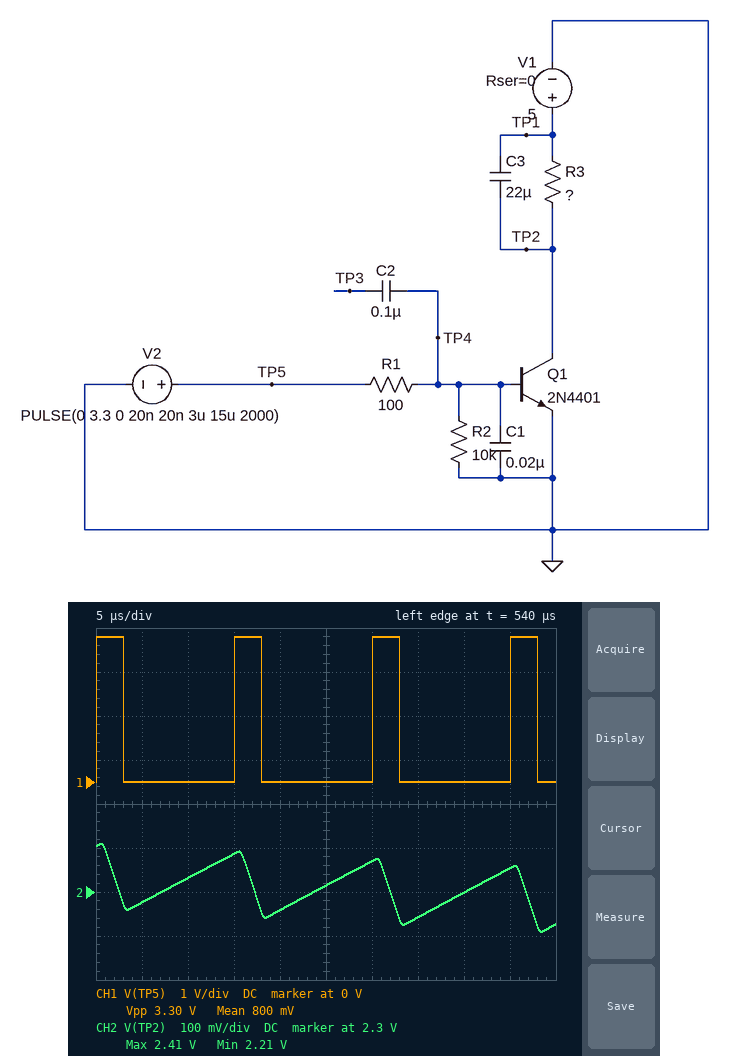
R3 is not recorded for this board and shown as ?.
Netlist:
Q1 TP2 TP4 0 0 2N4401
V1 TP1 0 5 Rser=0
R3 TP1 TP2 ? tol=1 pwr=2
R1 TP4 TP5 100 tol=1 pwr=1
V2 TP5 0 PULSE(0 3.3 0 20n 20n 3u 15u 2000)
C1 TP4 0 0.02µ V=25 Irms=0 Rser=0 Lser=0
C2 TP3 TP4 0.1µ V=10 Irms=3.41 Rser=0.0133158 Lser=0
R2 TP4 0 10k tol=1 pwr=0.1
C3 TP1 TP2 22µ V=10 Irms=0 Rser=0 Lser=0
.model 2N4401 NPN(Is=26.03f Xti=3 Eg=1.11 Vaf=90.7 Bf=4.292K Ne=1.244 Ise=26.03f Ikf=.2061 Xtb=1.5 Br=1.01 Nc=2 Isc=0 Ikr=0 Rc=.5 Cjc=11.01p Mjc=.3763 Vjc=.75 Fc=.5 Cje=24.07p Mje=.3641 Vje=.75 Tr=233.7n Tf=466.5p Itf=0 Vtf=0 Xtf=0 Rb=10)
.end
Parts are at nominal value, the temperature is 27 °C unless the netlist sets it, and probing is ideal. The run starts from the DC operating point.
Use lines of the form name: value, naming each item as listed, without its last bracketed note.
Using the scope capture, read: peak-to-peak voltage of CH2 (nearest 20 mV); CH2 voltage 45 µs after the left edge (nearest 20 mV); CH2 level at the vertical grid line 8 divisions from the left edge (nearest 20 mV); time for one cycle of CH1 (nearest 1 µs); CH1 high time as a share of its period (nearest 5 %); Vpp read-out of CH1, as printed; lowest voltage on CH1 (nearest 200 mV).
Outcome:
peak-to-peak voltage of CH2: 200 mV
CH2 voltage 45 µs after the left edge: 2.36 V
CH2 level at the vertical grid line 8 divisions from the left edge: 2.30 V
time for one cycle of CH1: 15 µs
CH1 high time as a share of its period: 20 %
Vpp read-out of CH1, as printed: 3.30 V
lowest voltage on CH1: 0 V
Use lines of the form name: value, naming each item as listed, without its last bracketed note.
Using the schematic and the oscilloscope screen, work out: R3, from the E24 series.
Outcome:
R3, from the E24 series: 11 Ω
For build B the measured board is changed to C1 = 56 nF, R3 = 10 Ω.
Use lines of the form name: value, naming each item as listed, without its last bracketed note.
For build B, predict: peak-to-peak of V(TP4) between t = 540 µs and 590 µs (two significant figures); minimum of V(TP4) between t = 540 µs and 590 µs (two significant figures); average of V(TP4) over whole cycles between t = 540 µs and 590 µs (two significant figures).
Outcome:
peak-to-peak of V(TP4) between t = 540 µs and 590 µs: 970 mV
minimum of V(TP4) between t = 540 µs and 590 µs: 110 mV
average of V(TP4) over whole cycles between t = 540 µs and 590 µs: 460 mV
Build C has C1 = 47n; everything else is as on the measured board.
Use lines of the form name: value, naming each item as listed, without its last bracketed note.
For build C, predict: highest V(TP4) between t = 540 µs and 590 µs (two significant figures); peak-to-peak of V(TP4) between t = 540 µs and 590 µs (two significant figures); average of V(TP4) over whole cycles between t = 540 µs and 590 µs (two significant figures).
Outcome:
highest V(TP4) between t = 540 µs and 590 µs: 1.1 V
peak-to-peak of V(TP4) between t = 540 µs and 590 µs: 1.0 V
average of V(TP4) over whole cycles between t = 540 µs and 590 µs: 430 mV
